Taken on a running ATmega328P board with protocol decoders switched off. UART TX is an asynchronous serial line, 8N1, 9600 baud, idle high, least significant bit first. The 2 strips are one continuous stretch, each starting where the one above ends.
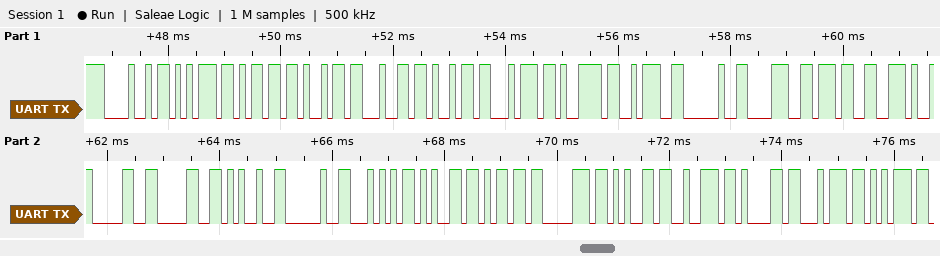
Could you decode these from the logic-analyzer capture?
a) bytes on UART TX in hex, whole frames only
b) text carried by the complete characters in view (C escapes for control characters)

48 75 6D 69 64 69 74 79 3A 20 38 37 2E 30 30 25 20 54 65 6D 70 65 72 61 74 75
"Humidity: 87.00% Temperatu"
